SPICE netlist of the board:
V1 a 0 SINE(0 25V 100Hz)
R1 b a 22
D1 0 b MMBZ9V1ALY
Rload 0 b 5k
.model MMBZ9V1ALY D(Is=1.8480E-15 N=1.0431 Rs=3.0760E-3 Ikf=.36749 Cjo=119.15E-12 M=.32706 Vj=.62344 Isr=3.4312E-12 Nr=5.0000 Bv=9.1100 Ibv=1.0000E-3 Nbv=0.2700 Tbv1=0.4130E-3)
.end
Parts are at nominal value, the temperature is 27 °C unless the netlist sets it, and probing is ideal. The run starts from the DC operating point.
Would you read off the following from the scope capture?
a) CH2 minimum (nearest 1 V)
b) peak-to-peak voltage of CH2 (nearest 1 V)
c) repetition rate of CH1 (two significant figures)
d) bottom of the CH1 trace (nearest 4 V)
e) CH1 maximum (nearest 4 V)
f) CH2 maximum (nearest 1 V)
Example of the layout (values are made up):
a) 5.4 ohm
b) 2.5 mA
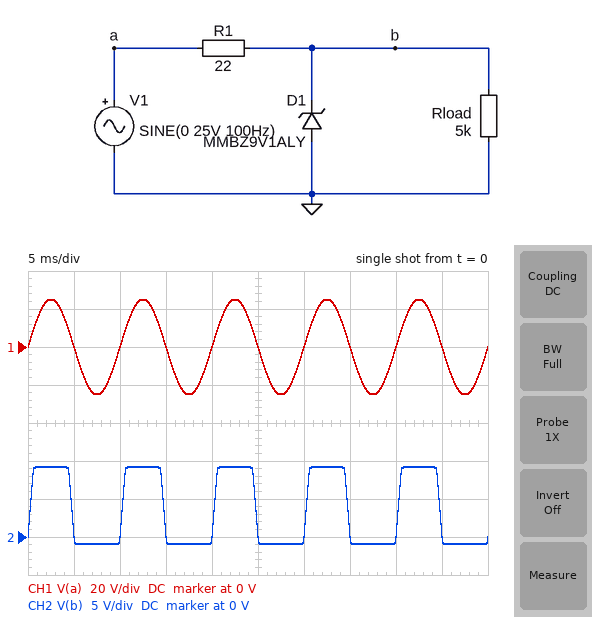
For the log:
a) -1 V
b) 10 V
c) 100 Hz
d) -24 V
e) 24 V
f) 9 V
